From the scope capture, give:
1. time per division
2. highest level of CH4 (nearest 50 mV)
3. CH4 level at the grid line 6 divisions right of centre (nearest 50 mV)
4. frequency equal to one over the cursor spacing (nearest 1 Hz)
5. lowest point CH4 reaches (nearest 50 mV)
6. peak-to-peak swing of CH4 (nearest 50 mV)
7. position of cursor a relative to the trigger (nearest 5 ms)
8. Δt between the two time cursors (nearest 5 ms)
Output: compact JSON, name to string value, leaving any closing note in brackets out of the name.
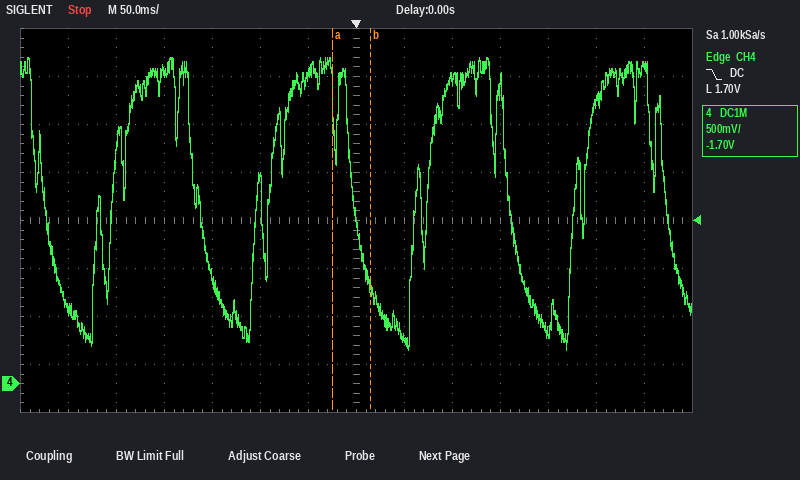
{"time per division": "50 ms", "highest level of CH4": "3.40 V", "CH4 level at the grid line 6 divisions right of centre": "3.30 V", "frequency equal to one over the cursor spacing": "25 Hz", "lowest point CH4 reaches": "350 mV", "peak-to-peak swing of CH4": "3.05 V", "position of cursor a relative to the trigger": "-25 ms", "Δt between the two time cursors": "40 ms"}
